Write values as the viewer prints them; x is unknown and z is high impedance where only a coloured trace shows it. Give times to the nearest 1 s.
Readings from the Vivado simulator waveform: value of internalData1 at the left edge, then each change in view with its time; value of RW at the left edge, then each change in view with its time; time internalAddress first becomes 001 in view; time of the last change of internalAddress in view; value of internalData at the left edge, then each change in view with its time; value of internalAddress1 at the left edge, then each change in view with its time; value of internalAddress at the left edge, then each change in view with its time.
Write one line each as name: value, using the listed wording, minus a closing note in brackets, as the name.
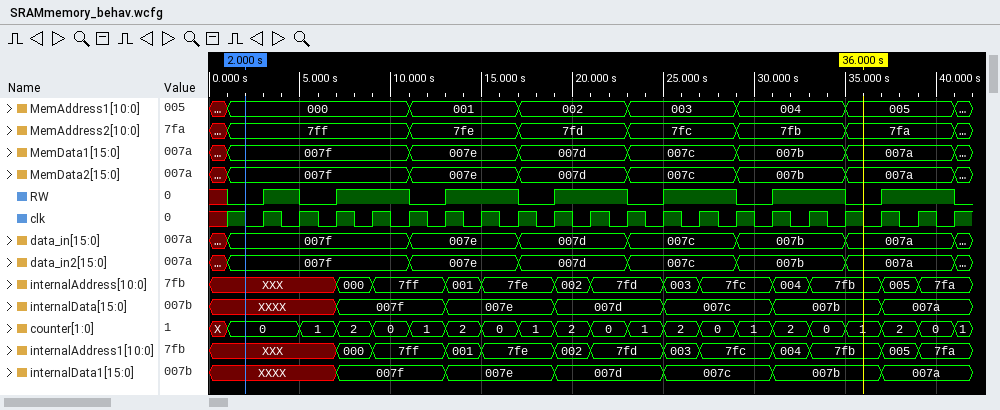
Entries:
value of internalData1 at the left edge, then each change in view with its time: XXXX, 007f at 7 s, 007e at 13 s, 007d at 19 s, 007c at 25 s, 007b at 31 s, 007a at 37 s
value of RW at the left edge, then each change in view with its time: x, 0 at 1 s, 1 at 3 s, 0 at 5 s, 1 at 7 s, 0 at 11 s, 1 at 13 s, 0 at 17 s, 1 at 19 s, 0 at 23 s, 1 at 25 s, 0 at 29 s, 1 at 31 s, 0 at 35 s, 1 at 37 s, 0 at 41 s
time internalAddress first becomes 001 in view: 13 s
time of the last change of internalAddress in view: 39 s
value of internalData at the left edge, then each change in view with its time: XXXX, 007f at 7 s, 007e at 13 s, 007d at 19 s, 007c at 25 s, 007b at 31 s, 007a at 37 s
value of internalAddress1 at the left edge, then each change in view with its time: XXX, 000 at 7 s, 7ff at 9 s, 001 at 13 s, 7fe at 15 s, 002 at 19 s, 7fd at 21 s, 003 at 25 s, 7fc at 27 s, 004 at 31 s, 7fb at 33 s, 005 at 37 s, 7fa at 39 s
value of internalAddress at the left edge, then each change in view with its time: XXX, 000 at 7 s, 7ff at 9 s, 001 at 13 s, 7fe at 15 s, 002 at 19 s, 7fd at 21 s, 003 at 25 s, 7fc at 27 s, 004 at 31 s, 7fb at 33 s, 005 at 37 s, 7fa at 39 s
